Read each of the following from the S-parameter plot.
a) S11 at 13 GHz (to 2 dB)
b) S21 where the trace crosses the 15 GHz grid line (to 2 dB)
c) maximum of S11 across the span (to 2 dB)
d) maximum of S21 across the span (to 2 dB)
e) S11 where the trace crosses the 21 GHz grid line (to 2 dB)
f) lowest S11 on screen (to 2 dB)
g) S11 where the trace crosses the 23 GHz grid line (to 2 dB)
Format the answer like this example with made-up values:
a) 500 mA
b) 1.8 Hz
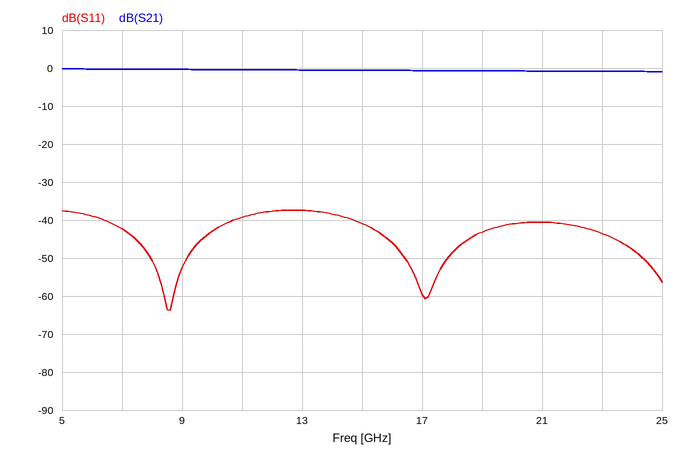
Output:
a) -38 dB
b) 0 dB
c) -38 dB
d) 0 dB
e) -40 dB
f) -64 dB
g) -44 dB
